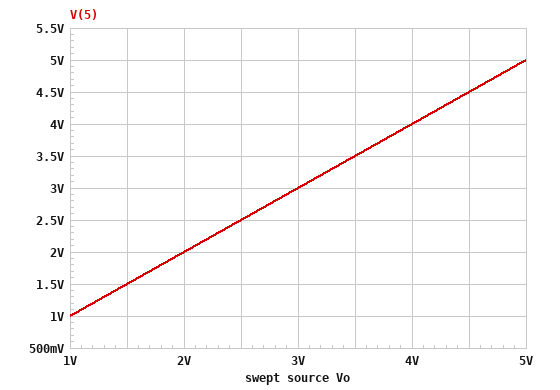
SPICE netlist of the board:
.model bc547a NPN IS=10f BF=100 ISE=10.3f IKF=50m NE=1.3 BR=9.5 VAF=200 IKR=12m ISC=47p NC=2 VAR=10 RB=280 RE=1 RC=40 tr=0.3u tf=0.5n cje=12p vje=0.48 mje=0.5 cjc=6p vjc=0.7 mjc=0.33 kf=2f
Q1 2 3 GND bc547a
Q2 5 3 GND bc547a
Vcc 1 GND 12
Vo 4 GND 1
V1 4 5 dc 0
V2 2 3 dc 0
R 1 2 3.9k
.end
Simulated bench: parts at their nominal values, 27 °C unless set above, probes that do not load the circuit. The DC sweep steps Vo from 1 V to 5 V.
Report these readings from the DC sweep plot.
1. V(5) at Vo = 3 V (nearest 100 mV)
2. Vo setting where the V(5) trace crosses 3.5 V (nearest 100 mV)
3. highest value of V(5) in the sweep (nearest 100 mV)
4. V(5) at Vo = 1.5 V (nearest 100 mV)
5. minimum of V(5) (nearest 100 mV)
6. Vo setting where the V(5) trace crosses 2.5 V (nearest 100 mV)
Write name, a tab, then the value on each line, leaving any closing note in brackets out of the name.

V(5) at Vo = 3 V	3.0 V
Vo setting where the V(5) trace crosses 3.5 V	3.5 V
highest value of V(5) in the sweep	5.0 V
V(5) at Vo = 1.5 V	1.5 V
minimum of V(5)	1.0 V
Vo setting where the V(5) trace crosses 2.5 V	2.5 V
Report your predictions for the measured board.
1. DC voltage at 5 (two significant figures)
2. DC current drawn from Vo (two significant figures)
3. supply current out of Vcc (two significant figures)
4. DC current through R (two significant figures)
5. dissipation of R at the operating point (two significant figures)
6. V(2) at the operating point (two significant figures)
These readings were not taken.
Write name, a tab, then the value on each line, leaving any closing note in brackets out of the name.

DC voltage at 5	1.0 V
DC current drawn from Vo	2.8 mA
supply current out of Vcc	2.9 mA
DC current through R	2.9 mA
dissipation of R at the operating point	33 mW
V(2) at the operating point	700 mV
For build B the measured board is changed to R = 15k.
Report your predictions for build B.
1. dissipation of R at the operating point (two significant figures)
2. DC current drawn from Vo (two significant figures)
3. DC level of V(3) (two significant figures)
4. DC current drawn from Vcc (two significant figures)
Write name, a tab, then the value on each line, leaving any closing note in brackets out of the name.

dissipation of R at the operating point	8.6 mW
DC current drawn from Vo	740 µA
DC level of V(3)	650 mV
DC current drawn from Vcc	760 µA
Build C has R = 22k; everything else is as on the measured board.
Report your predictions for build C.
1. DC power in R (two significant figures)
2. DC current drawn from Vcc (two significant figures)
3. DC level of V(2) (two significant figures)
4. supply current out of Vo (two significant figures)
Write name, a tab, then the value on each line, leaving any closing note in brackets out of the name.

DC power in R	5.9 mW
DC current drawn from Vcc	520 µA
DC level of V(2)	640 mV
supply current out of Vo	500 µA
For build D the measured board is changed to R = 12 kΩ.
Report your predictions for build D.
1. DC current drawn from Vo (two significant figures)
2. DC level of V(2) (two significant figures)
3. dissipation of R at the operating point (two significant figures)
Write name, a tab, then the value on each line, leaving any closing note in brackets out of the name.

DC current drawn from Vo	920 µA
DC level of V(2)	660 mV
dissipation of R at the operating point	11 mW
